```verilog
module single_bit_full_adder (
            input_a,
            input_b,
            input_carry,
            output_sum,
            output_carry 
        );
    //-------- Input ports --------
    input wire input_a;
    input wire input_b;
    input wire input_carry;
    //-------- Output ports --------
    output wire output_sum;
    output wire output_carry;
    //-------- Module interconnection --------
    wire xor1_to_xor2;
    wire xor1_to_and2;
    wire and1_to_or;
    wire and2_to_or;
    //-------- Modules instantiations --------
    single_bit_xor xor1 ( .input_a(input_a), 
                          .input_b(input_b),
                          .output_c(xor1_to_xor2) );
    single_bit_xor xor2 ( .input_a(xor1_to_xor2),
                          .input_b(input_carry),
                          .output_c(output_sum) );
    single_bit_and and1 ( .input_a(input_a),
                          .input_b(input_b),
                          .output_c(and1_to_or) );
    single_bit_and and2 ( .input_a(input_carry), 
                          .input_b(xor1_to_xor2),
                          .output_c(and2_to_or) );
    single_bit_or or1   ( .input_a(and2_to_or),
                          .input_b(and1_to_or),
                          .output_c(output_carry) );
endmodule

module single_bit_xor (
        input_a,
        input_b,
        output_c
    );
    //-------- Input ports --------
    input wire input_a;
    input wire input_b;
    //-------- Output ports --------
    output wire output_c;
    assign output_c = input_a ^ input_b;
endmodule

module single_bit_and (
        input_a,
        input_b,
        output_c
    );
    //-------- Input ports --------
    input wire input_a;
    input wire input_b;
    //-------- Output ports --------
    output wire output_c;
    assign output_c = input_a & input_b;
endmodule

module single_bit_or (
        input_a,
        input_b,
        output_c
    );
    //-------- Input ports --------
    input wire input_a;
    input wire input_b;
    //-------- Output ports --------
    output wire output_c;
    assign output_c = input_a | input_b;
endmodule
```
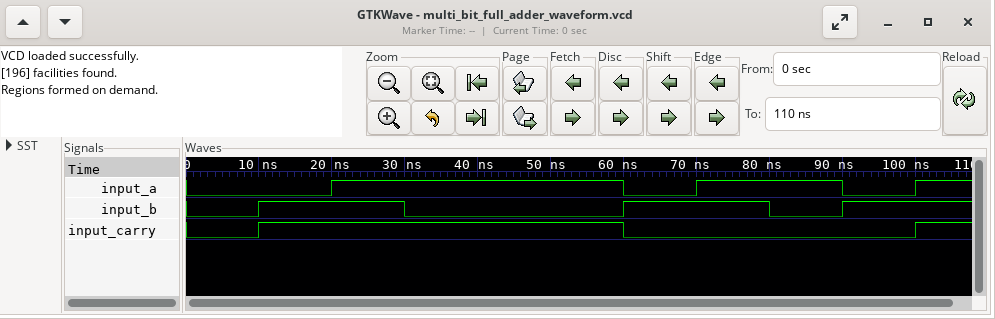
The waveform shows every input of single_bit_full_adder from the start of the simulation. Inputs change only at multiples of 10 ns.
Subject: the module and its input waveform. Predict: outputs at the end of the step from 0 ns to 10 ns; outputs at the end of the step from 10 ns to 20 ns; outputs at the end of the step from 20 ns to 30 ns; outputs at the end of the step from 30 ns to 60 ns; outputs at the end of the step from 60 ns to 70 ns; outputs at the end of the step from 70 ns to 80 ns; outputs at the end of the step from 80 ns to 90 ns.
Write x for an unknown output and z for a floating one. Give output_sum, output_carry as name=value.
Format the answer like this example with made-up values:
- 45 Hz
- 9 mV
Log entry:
- output_sum=0, output_carry=0
- output_sum=0, output_carry=1
- output_sum=1, output_carry=1
- output_sum=0, output_carry=1
- output_sum=1, output_carry=0
- output_sum=0, output_carry=1
- output_sum=1, output_carry=0
